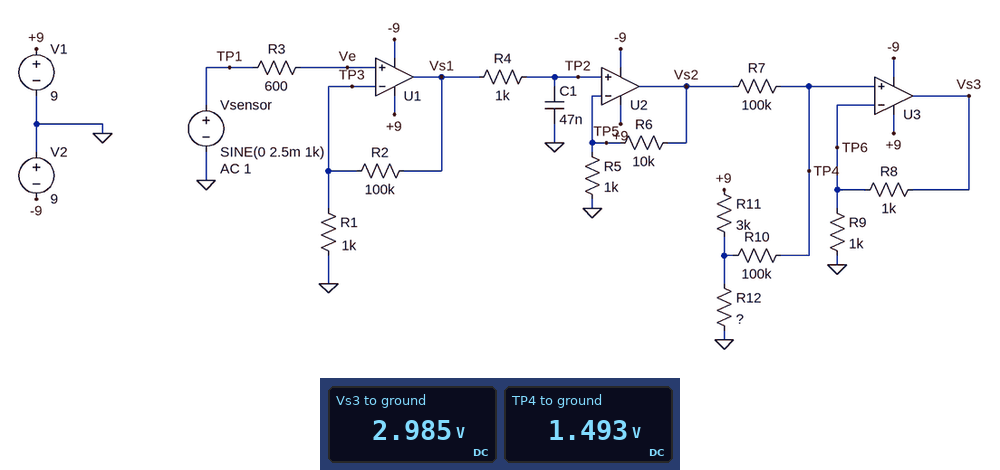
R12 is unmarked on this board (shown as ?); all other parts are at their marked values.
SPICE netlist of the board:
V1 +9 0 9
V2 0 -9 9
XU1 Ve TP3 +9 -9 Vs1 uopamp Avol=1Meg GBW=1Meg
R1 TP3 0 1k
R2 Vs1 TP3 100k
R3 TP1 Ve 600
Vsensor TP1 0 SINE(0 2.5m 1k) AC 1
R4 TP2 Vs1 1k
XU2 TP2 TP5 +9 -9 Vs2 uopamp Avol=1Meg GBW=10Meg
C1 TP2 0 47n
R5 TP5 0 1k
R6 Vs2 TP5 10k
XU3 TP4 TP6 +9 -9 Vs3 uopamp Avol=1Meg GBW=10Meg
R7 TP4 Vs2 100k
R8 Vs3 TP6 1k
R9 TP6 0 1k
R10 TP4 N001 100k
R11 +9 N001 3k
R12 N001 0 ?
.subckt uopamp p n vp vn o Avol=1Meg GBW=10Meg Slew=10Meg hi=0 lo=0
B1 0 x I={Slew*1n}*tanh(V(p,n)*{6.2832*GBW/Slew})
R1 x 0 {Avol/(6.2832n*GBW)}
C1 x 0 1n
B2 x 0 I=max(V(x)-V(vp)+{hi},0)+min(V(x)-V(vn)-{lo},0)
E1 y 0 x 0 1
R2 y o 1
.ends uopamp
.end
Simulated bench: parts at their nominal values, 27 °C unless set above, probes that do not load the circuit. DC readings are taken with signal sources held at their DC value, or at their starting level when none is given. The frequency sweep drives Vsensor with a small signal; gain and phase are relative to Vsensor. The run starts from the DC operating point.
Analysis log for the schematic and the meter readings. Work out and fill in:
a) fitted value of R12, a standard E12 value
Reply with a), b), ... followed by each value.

a) 1.5 kΩ
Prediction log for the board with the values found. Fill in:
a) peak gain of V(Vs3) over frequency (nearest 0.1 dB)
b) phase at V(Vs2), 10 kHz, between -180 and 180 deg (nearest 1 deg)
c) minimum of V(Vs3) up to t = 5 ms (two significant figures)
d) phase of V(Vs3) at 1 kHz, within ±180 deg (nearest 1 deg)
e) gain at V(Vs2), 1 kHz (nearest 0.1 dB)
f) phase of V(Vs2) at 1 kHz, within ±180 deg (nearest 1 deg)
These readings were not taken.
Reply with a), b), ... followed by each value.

a) 61.0 dB
b) -117 deg
c) 320 mV
d) -22 deg
e) 60.5 dB
f) -22 deg
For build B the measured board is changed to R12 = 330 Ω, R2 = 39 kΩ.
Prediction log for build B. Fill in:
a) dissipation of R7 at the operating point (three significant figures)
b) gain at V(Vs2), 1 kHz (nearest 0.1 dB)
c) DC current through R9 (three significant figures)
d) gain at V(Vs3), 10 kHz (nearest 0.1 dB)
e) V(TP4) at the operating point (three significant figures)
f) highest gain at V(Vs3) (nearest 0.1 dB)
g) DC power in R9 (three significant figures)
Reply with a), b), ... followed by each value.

a) 1.98 µW
b) 52.5 dB
c) 445 µA
d) 42.4 dB
e) 445 mV
f) 52.9 dB
g) 198 µW
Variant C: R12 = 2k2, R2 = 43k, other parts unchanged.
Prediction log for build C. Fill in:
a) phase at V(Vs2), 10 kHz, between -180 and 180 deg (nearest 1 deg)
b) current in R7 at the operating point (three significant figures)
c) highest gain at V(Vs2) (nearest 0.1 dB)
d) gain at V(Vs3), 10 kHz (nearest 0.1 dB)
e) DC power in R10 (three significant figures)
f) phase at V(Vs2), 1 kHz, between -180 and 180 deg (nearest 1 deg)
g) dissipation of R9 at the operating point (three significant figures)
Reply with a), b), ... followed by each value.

a) -96 deg
b) 18.9 µA
c) 53.7 dB
d) 43.1 dB
e) 35.8 µW
f) -19 deg
g) 3.58 mW
